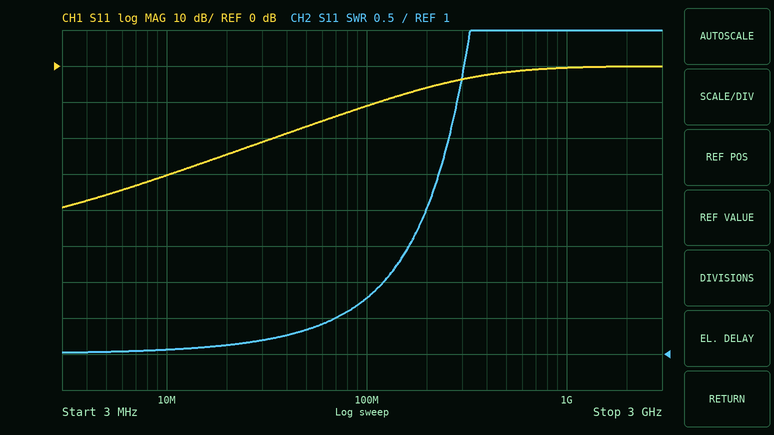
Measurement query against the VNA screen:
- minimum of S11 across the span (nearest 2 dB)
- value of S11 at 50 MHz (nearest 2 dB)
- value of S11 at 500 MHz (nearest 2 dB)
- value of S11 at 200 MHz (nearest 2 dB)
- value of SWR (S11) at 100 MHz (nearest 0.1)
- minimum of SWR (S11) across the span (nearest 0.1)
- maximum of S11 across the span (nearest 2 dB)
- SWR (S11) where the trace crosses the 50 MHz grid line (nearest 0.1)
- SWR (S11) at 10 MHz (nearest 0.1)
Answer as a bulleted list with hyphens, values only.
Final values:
- -40 dB
- -16 dB
- -2 dB
- -6 dB
- 1.8
- 1.0
- 0 dB
- 1.3
- 1.1
